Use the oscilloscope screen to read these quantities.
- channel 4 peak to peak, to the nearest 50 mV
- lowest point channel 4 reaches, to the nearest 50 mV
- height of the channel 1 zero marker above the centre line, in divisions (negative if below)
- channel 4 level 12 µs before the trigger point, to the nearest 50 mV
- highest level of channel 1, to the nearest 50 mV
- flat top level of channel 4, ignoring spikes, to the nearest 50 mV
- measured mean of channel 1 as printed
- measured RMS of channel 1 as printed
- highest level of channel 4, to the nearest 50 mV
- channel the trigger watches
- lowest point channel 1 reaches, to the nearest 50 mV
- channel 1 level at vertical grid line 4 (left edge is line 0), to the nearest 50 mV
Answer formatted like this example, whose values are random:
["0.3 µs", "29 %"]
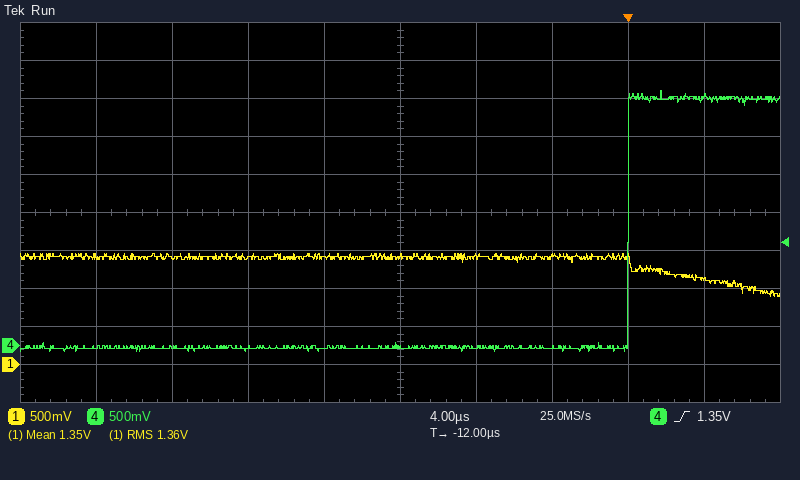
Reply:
["3.45 V", "-100 mV", "-4.0 div", "0 mV", "1.45 V", "3.25 V", "1.35 V", "1.36 V", "3.35 V", "channel 4", "900 mV", "1.40 V"]
